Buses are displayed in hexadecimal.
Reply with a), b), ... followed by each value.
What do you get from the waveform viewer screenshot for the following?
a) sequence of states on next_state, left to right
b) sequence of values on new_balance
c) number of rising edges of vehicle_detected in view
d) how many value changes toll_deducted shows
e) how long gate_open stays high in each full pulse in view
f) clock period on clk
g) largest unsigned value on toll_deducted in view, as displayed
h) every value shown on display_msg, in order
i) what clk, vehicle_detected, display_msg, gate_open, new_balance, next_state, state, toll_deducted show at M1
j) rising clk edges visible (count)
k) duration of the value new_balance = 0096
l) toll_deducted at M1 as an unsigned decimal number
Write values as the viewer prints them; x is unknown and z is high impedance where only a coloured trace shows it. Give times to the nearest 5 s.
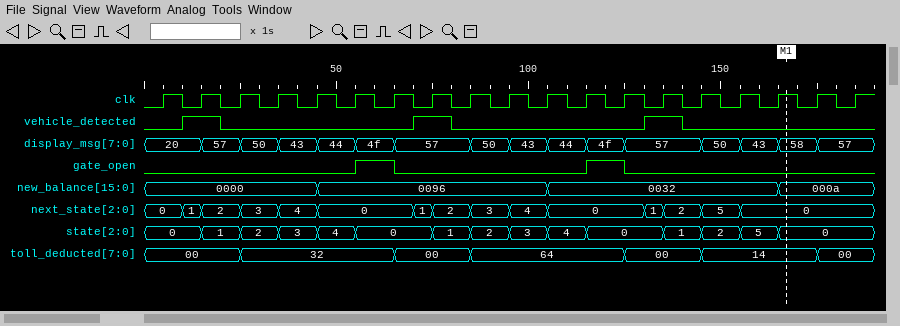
a) 0, 1, 2, 3, 4, 0, 1, 2, 3, 4, 0, 1, 2, 5, 0
b) 0000, 0096, 0032, 000a
c) 3
d) 6
e) 10 s, 10 s
f) 10 s
g) 64
h) 20, 57, 50, 43, 44, 4f, 57, 50, 43, 44, 4f, 57, 50, 43, 58, 57
i) clk=1, vehicle_detected=0, display_msg=58, gate_open=0, new_balance=000a, next_state=0, state=0, toll_deducted=14
j) 19
k) 60 s
l) 20
